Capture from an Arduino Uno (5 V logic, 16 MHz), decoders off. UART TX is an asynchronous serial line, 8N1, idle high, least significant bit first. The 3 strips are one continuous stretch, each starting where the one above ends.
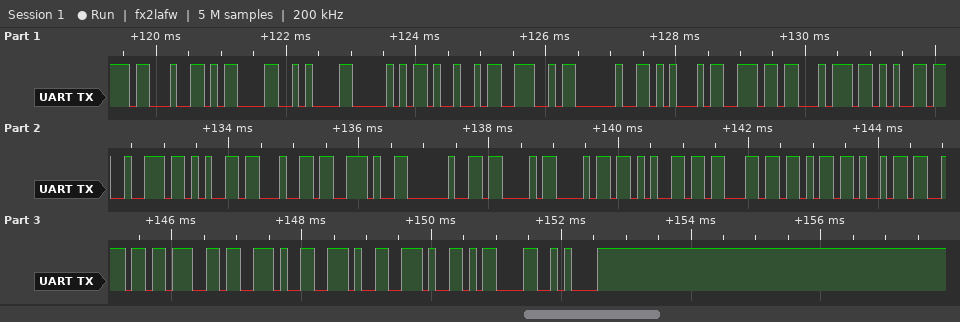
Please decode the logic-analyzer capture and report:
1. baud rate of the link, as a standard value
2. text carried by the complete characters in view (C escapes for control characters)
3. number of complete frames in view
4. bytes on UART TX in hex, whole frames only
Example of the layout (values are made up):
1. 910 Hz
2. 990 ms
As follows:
1. 9600 baud
2. "#\r\nPIN Entered. Checking...\r\n"
3. 29
4. 23 0D 0A 50 49 4E 20 45 6E 74 65 72 65 64 2E 20 43 68 65 63 6B 69 6E 67 2E 2E 2E 0D 0A
